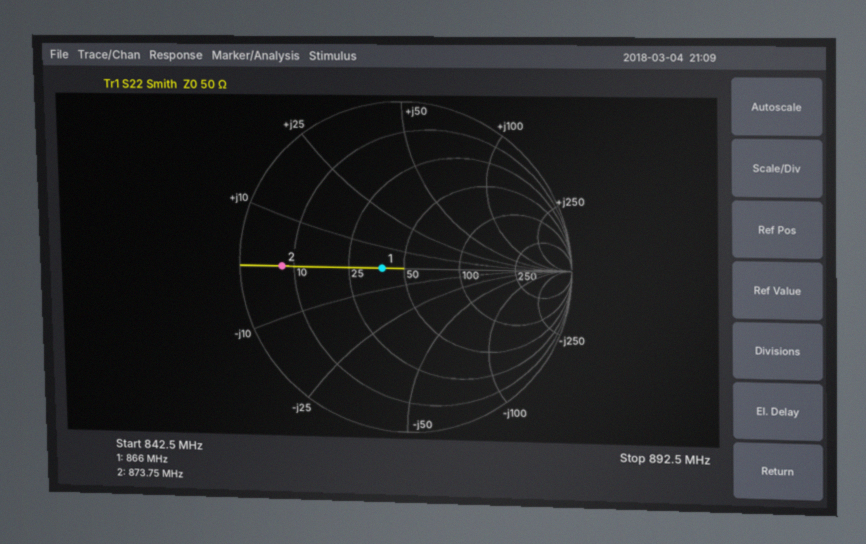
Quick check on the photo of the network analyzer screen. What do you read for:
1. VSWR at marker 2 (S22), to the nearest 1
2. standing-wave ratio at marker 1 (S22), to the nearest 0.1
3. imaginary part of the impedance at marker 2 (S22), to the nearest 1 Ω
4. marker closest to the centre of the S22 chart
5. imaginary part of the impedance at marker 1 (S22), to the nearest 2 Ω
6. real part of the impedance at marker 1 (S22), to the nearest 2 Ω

7
1.3
0 Ω
marker 1
0 Ω
38 Ω
